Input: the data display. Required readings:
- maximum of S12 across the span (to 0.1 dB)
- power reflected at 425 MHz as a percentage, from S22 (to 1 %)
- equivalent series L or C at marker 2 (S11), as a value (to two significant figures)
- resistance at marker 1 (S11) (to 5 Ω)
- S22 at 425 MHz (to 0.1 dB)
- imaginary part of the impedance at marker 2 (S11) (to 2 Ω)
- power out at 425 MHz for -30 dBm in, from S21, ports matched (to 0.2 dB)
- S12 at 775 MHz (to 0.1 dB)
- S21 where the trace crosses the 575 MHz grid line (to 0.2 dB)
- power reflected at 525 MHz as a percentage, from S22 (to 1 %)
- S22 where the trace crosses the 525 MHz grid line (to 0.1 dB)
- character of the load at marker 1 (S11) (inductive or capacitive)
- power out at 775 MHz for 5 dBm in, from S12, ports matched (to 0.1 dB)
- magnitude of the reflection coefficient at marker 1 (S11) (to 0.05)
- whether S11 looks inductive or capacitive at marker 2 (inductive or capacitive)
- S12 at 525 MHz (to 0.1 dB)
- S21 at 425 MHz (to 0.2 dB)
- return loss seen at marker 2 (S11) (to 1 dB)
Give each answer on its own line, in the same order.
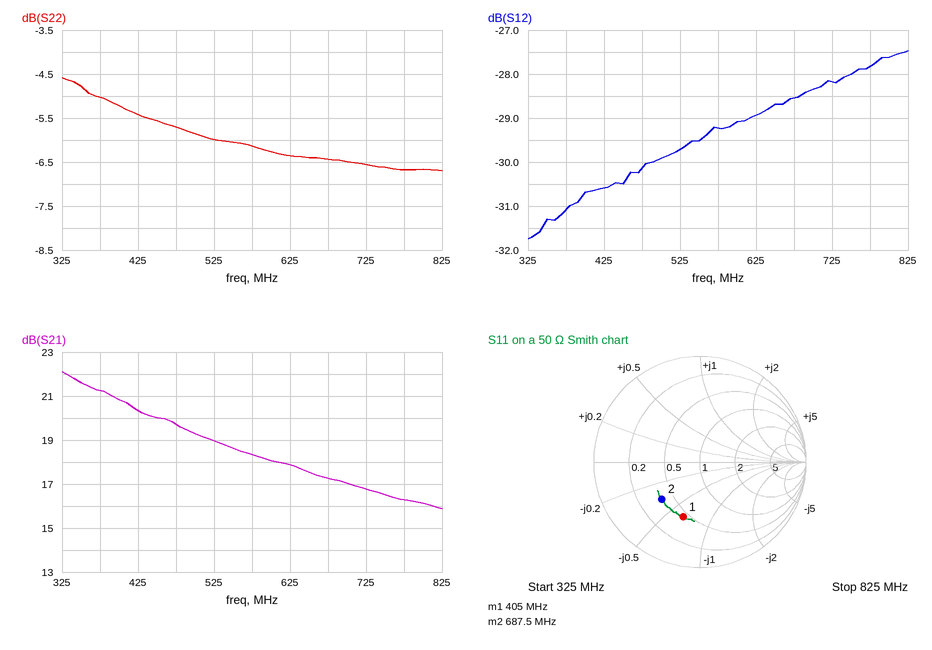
-27.5 dB
29 %
13 pF
20 Ω
-5.4 dB
-18 Ω
-9.6 dBm
-27.8 dB
18.4 dB
25 %
-6.0 dB
capacitive
-22.8 dBm
0.55
capacitive
-29.7 dB
20.4 dB
6 dB
